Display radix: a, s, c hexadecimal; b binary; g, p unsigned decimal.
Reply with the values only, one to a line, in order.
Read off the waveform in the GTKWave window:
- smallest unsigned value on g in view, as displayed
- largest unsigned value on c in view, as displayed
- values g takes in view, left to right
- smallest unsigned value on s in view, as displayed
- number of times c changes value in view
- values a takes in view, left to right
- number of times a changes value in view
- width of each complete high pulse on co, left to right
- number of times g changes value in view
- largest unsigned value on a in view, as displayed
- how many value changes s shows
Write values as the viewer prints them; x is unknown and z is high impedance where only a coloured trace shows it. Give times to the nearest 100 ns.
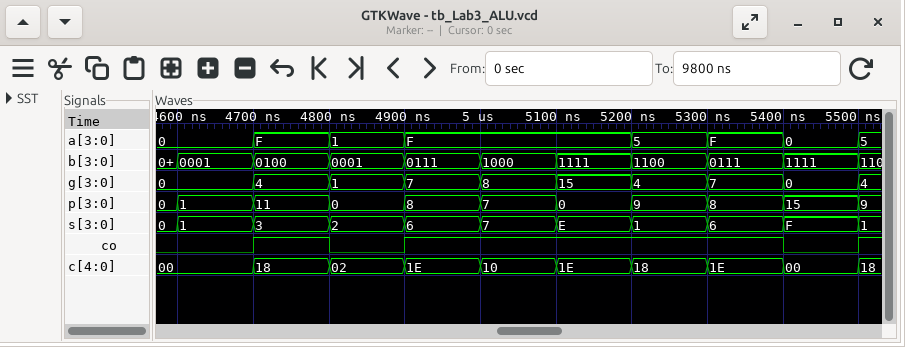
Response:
0
1E
0, 4, 1, 7, 8, 15, 4, 7, 0, 4
0
9
0, F, 1, F, 5, F, 0, 5
7
100 ns, 500 ns
9
F
10
